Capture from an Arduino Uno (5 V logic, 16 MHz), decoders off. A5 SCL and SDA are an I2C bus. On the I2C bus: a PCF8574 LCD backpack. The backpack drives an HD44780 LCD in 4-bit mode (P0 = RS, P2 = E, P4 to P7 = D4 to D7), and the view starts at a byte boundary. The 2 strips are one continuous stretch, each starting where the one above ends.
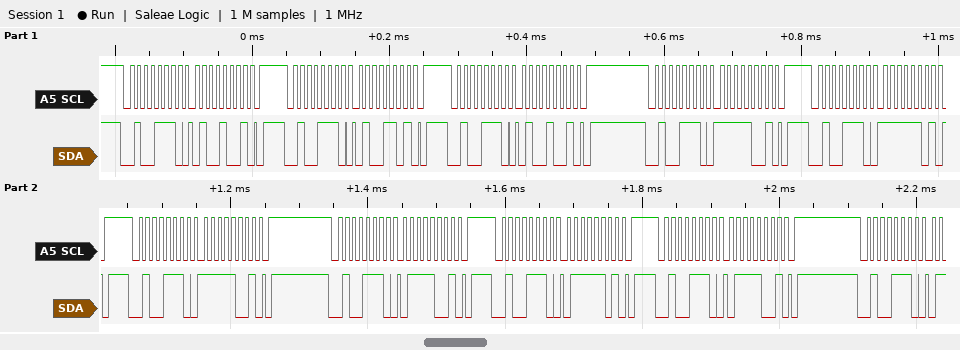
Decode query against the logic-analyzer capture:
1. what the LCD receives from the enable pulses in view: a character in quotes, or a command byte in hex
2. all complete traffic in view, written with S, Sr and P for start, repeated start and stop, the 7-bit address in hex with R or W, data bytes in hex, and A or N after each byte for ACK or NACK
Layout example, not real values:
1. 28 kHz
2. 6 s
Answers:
1. 'O'
2. S 27W A 49 A P S 27W A 4D A P S 27W A 49 A P S 27W A F9 A P S 27W A FD A P S 27W A F9 A P S 27W A 79 A P S 27W A 7D A P S 27W A 79 A P S 27W A
